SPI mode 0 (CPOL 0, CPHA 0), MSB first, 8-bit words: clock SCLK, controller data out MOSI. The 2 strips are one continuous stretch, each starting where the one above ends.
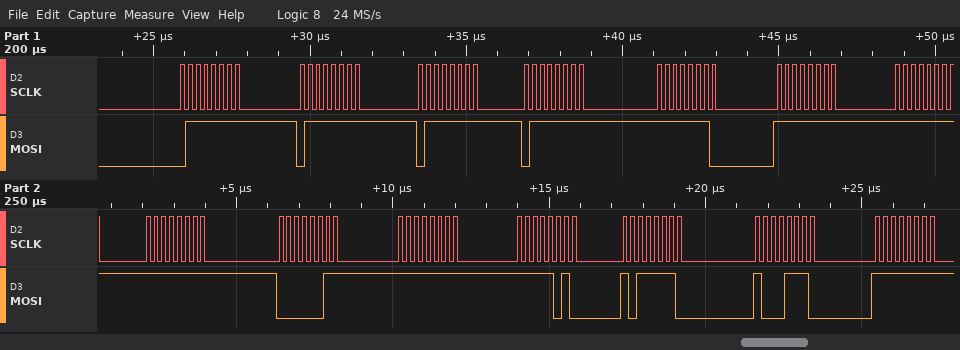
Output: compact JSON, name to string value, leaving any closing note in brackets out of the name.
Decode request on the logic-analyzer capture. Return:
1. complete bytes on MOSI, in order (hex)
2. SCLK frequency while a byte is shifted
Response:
{"complete bytes on MOSI, in order": "7F 7F 7F 7F FE FF FF FF 03 FF FA BE 8E FF", "SCLK frequency while a byte is shifted": "4 MHz"}
